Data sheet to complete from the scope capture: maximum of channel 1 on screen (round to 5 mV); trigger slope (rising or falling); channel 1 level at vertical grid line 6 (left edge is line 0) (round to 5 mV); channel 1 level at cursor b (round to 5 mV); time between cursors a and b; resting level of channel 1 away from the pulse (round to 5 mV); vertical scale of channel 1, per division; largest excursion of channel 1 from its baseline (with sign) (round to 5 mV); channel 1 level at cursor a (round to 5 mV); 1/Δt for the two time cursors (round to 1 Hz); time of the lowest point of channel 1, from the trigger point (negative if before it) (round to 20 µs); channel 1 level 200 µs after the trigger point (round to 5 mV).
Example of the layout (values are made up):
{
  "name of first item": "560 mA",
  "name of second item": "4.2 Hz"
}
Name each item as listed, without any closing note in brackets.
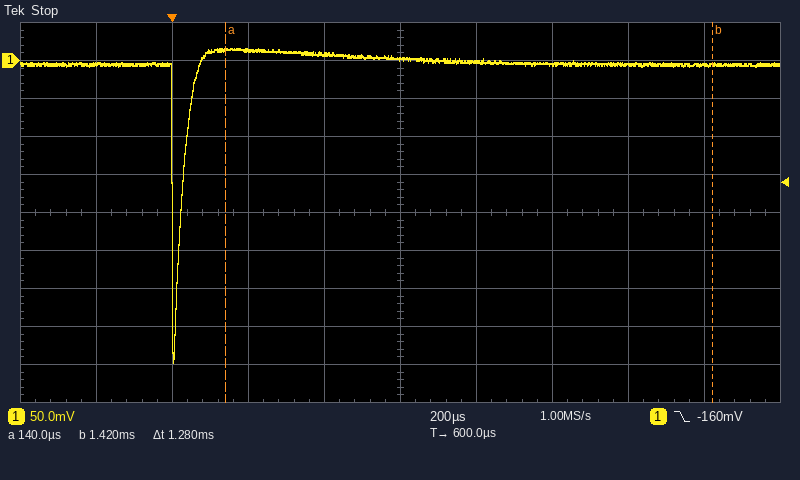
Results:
{
  "maximum of channel 1 on screen": "15 mV",
  "trigger slope": "falling",
  "channel 1 level at vertical grid line 6 (left edge is line 0)": "0 mV",
  "channel 1 level at cursor b": "-5 mV",
  "time between cursors a and b": "1.28 ms",
  "resting level of channel 1 away from the pulse": "-5 mV",
  "vertical scale of channel 1, per division": "50 mV",
  "largest excursion of channel 1 from its baseline (with sign)": "-395 mV",
  "channel 1 level at cursor a": "15 mV",
  "1/Δt for the two time cursors": "781 Hz",
  "time of the lowest point of channel 1, from the trigger point (negative if before it)": "0 µs",
  "channel 1 level 200 µs after the trigger point": "15 mV"
}
